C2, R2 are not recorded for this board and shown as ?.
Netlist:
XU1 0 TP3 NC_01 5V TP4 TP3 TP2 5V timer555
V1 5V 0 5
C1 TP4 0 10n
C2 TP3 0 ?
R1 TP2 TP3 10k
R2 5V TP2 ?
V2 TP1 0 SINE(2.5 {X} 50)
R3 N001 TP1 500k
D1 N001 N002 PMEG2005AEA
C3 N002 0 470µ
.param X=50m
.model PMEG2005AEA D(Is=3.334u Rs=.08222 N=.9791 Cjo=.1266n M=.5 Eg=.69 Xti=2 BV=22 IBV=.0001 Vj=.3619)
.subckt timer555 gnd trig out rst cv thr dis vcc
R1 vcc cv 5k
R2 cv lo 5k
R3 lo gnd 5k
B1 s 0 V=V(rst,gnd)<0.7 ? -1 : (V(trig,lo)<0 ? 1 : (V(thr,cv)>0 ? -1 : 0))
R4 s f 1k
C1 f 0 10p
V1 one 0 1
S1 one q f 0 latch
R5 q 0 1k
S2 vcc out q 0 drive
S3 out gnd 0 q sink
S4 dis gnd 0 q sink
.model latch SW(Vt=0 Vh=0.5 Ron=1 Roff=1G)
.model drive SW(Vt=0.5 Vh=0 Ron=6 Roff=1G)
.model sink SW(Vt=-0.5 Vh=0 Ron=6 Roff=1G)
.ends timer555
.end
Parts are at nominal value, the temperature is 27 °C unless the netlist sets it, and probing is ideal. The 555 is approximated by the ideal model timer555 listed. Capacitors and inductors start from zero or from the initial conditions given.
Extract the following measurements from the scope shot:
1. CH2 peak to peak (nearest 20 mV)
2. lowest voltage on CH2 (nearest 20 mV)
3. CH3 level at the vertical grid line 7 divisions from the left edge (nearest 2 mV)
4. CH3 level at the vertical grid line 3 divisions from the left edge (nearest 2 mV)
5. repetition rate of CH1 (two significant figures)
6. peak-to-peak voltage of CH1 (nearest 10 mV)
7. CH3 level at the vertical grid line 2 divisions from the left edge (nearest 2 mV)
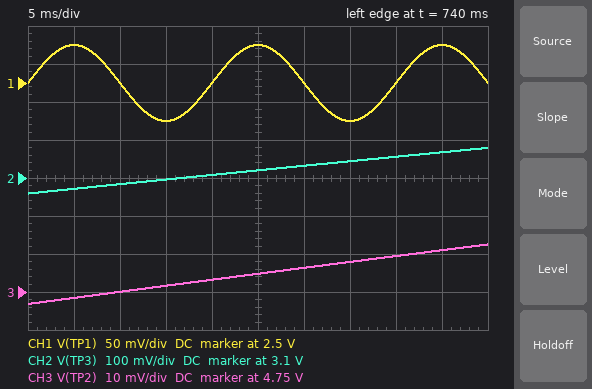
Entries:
120 mV
3.06 V
4.758 V
4.752 V
50 Hz
100 mV
4.750 V
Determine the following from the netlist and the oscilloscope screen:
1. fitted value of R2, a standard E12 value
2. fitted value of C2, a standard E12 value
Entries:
1.5 kΩ
68 µF
